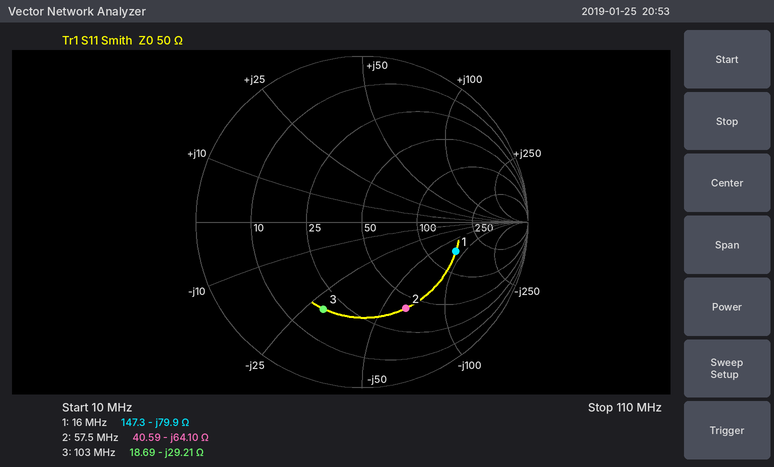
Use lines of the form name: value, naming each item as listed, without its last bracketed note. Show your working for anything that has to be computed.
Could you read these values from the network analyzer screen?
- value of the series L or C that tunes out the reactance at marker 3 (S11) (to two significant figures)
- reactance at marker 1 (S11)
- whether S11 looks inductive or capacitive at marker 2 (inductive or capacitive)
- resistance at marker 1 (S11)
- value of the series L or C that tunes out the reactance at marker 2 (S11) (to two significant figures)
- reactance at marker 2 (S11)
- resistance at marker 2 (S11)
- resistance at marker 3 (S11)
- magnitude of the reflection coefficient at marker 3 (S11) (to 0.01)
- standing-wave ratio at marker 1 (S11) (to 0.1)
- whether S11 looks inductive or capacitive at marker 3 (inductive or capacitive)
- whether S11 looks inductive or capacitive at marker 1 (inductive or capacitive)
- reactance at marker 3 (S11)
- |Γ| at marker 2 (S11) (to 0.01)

value of the series L or C that tunes out the reactance at marker 3 (S11): L = 29.21 Ω/(2π × 103 MHz) ≈ 45 nH
reactance at marker 1: -79.9 Ω
whether S11 looks inductive or capacitive at marker 2: capacitive
resistance at marker 1: 147.3 Ω
value of the series L or C that tunes out the reactance at marker 2 (S11): L = 64.1 Ω/(2π × 57.5 MHz) ≈ 177 nH, so 180 nH to two significant figures
reactance at marker 2: -64.10 Ω
resistance at marker 2: 40.59 Ω
resistance at marker 3: 18.69 Ω
magnitude of the reflection coefficient at marker 3 (S11): 0.57
standing-wave ratio at marker 1 (S11): 3.9
whether S11 looks inductive or capacitive at marker 3: capacitive
whether S11 looks inductive or capacitive at marker 1: capacitive
reactance at marker 3: -29.21 Ω
|Γ| at marker 2 (S11): 0.58
